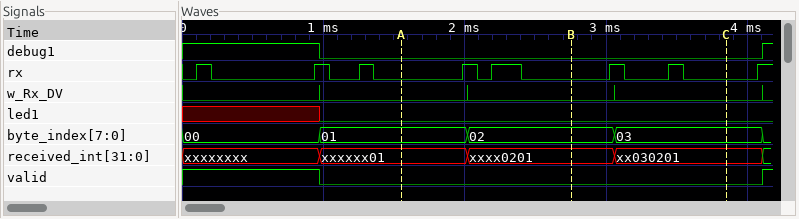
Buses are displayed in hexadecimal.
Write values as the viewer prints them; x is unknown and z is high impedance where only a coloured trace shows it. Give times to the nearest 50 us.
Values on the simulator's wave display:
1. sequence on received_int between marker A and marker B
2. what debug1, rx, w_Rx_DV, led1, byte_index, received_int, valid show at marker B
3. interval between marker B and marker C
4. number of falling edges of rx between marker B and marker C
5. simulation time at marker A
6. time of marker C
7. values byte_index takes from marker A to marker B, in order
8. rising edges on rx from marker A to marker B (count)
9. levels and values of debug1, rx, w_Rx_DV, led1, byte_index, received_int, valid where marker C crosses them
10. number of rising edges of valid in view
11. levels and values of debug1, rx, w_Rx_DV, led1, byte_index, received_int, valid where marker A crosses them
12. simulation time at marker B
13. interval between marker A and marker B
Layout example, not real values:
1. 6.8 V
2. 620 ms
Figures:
1. xxxxxx01, xxxx0201
2. debug1=0, rx=0, w_Rx_DV=0, led1=0, byte_index=02, received_int=xxxx0201, valid=0
3. 1100 us
4. 2
5. 1550 us
6. 3850 us
7. 01, 02
8. 2
9. debug1=0, rx=0, w_Rx_DV=0, led1=0, byte_index=03, received_int=xx030201, valid=0
10. 1
11. debug1=0, rx=0, w_Rx_DV=0, led1=0, byte_index=01, received_int=xxxxxx01, valid=0
12. 2750 us
13. 1200 us
